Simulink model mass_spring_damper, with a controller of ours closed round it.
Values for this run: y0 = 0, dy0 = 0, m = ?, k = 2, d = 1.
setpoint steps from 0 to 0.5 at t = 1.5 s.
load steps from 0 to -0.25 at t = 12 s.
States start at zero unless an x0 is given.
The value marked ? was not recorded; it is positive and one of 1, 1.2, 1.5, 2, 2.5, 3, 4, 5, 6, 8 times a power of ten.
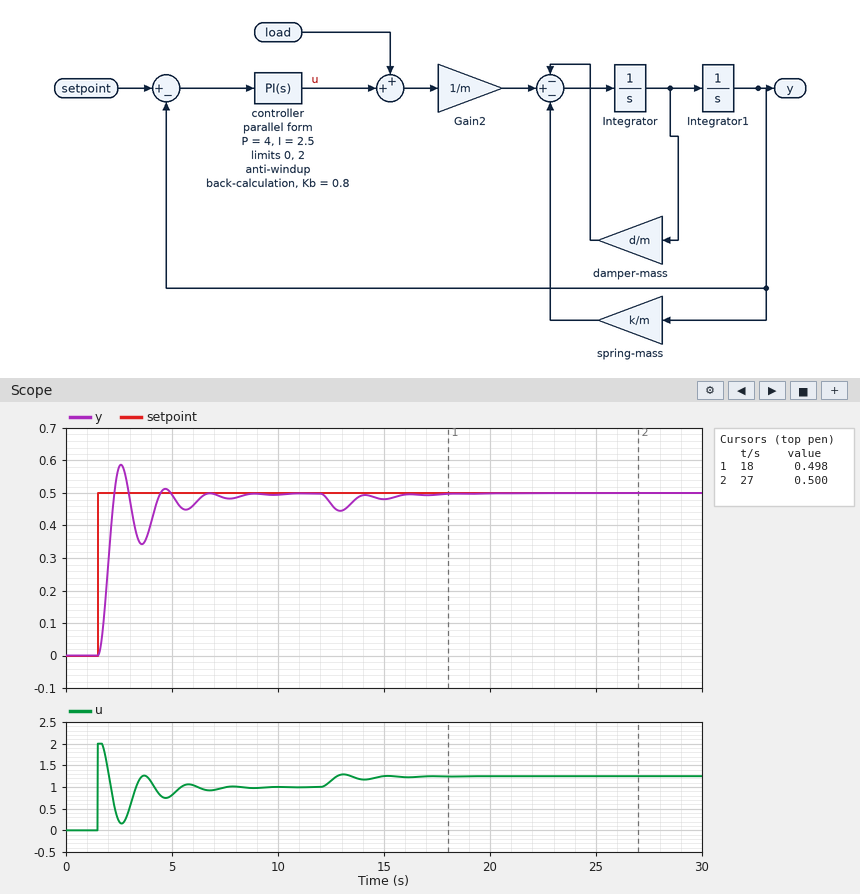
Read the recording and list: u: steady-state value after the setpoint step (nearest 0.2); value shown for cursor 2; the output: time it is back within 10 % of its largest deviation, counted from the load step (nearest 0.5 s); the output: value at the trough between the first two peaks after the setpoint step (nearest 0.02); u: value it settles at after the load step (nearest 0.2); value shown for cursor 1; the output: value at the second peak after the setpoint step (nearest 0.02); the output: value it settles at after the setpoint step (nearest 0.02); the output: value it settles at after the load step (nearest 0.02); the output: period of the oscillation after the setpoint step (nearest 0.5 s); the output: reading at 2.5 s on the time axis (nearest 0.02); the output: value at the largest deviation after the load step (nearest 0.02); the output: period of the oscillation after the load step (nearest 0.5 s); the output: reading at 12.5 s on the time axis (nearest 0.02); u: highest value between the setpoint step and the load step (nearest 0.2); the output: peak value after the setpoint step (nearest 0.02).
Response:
1.0
0.500
5.5 s
0.34
1.2
0.498
0.52
0.50
0.50
2.0 s
0.58
0.44
2.0 s
0.46
2.0
0.58
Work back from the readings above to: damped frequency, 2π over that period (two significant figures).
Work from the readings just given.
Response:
3.1 rad/s
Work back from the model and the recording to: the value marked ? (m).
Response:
0.6
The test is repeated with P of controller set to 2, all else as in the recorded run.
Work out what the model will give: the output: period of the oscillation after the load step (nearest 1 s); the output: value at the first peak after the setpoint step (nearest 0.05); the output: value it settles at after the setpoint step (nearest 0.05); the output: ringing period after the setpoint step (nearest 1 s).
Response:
3 s
0.55
0.50
3 s
